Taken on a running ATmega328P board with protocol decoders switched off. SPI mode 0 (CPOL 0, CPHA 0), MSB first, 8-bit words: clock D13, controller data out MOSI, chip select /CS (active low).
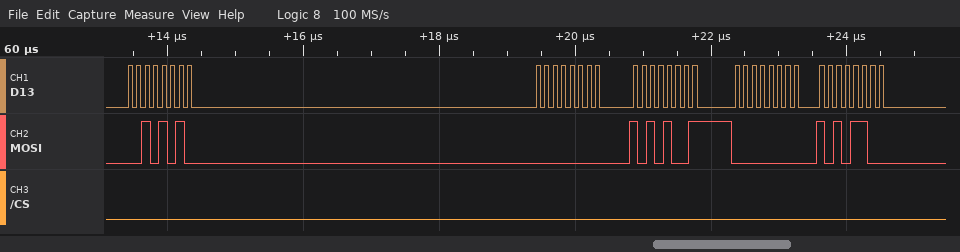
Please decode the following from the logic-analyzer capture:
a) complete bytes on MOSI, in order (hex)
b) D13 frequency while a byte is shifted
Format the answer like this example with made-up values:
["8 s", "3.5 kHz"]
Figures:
["2A 00 A9 00 AC", "8 MHz"]
